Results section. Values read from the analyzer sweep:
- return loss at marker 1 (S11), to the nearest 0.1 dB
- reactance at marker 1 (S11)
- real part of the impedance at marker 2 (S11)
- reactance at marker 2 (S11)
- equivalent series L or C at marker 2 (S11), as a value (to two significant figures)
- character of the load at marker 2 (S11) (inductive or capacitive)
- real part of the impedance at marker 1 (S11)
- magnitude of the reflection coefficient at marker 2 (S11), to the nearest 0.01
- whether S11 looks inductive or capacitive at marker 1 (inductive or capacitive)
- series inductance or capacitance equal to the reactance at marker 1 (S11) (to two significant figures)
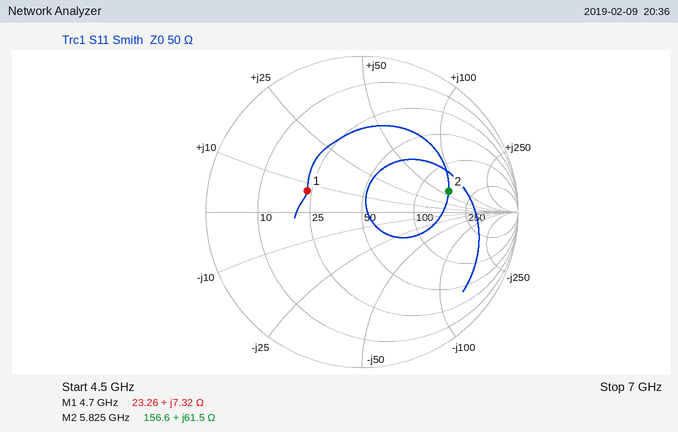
8.5 dB
+7.32 Ω
156.6 Ω
+61.5 Ω
1.7 nH
inductive
23.26 Ω
0.57
inductive
250 pH
